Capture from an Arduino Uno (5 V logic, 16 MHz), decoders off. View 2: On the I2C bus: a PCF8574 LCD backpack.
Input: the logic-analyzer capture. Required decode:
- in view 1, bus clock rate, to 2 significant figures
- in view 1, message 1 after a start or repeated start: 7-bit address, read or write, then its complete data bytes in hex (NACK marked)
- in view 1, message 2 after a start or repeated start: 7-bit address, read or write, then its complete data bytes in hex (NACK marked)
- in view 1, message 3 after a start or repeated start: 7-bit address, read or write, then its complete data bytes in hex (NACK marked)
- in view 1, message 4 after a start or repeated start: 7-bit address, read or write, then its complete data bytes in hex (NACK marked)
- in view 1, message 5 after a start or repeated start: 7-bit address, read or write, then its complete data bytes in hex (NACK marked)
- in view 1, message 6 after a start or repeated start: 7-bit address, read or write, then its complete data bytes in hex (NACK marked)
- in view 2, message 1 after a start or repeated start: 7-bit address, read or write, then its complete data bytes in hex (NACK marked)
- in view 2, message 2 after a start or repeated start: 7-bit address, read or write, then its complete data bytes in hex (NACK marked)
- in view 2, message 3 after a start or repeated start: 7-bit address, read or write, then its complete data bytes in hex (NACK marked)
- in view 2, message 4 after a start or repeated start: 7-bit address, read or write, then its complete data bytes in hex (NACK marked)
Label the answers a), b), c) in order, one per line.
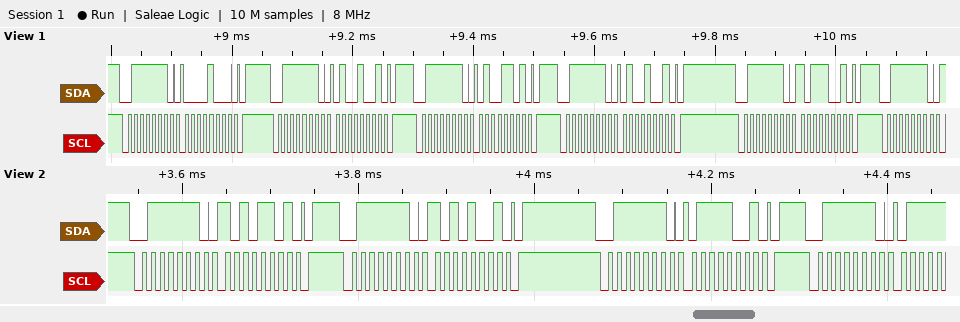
a) 100 kHz
b) 0x3F write: 08
c) 0x3F write: 49
d) 0x3F write: 4D
e) 0x3F write: 49
f) 0x3F write: B9
g) 0x3F write
h) 0x3F write: AD
i) 0x3F write: A9
j) 0x3F write: 79
k) 0x3F write
